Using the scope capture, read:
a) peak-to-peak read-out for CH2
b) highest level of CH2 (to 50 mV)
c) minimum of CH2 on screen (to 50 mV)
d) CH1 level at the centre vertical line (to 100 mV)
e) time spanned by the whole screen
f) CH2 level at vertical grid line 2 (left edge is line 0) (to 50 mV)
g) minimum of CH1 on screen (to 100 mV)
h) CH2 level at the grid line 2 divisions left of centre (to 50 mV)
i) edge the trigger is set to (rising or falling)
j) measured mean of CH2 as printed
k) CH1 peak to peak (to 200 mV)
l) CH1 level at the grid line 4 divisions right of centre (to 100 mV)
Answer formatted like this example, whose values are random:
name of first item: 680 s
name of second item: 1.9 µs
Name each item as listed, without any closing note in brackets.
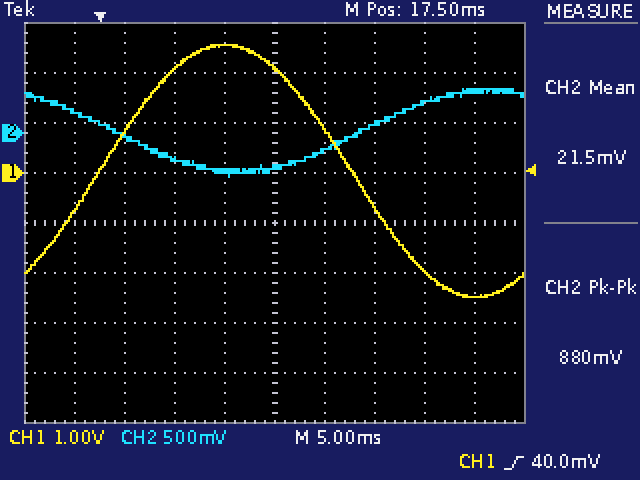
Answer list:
peak-to-peak read-out for CH2: 880 mV
highest level of CH2: 450 mV
minimum of CH2 on screen: -450 mV
CH1 level at the centre vertical line: 2.1 V
time spanned by the whole screen: 50 ms
CH2 level at vertical grid line 2 (left edge is line 0): -50 mV
minimum of CH1 on screen: -2.5 V
CH2 level at the grid line 2 divisions left of centre: -250 mV
edge the trigger is set to: rising
measured mean of CH2 as printed: 21.5 mV
CH1 peak to peak: 5.0 V
CH1 level at the grid line 4 divisions right of centre: -2.5 V
